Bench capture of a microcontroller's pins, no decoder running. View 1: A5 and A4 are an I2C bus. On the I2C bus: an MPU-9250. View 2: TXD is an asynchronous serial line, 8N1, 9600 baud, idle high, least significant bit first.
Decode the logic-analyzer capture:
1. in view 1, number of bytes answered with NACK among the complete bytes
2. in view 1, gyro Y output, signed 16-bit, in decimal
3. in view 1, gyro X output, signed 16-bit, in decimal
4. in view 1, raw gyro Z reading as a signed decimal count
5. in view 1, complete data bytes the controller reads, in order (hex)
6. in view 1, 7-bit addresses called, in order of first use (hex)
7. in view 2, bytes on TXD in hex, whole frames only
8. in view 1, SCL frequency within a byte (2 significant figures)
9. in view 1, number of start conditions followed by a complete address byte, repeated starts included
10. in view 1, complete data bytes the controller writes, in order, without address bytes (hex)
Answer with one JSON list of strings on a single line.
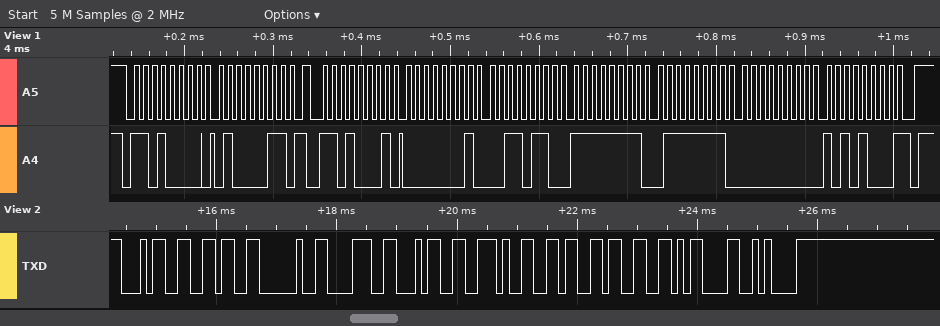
["1", "-129", "310", "168", "01 36 FF 7F 00 A8", "0x68", "34 36 20 38 34 2E 36 33 0D 0A", "100 kHz", "2", "43"]
